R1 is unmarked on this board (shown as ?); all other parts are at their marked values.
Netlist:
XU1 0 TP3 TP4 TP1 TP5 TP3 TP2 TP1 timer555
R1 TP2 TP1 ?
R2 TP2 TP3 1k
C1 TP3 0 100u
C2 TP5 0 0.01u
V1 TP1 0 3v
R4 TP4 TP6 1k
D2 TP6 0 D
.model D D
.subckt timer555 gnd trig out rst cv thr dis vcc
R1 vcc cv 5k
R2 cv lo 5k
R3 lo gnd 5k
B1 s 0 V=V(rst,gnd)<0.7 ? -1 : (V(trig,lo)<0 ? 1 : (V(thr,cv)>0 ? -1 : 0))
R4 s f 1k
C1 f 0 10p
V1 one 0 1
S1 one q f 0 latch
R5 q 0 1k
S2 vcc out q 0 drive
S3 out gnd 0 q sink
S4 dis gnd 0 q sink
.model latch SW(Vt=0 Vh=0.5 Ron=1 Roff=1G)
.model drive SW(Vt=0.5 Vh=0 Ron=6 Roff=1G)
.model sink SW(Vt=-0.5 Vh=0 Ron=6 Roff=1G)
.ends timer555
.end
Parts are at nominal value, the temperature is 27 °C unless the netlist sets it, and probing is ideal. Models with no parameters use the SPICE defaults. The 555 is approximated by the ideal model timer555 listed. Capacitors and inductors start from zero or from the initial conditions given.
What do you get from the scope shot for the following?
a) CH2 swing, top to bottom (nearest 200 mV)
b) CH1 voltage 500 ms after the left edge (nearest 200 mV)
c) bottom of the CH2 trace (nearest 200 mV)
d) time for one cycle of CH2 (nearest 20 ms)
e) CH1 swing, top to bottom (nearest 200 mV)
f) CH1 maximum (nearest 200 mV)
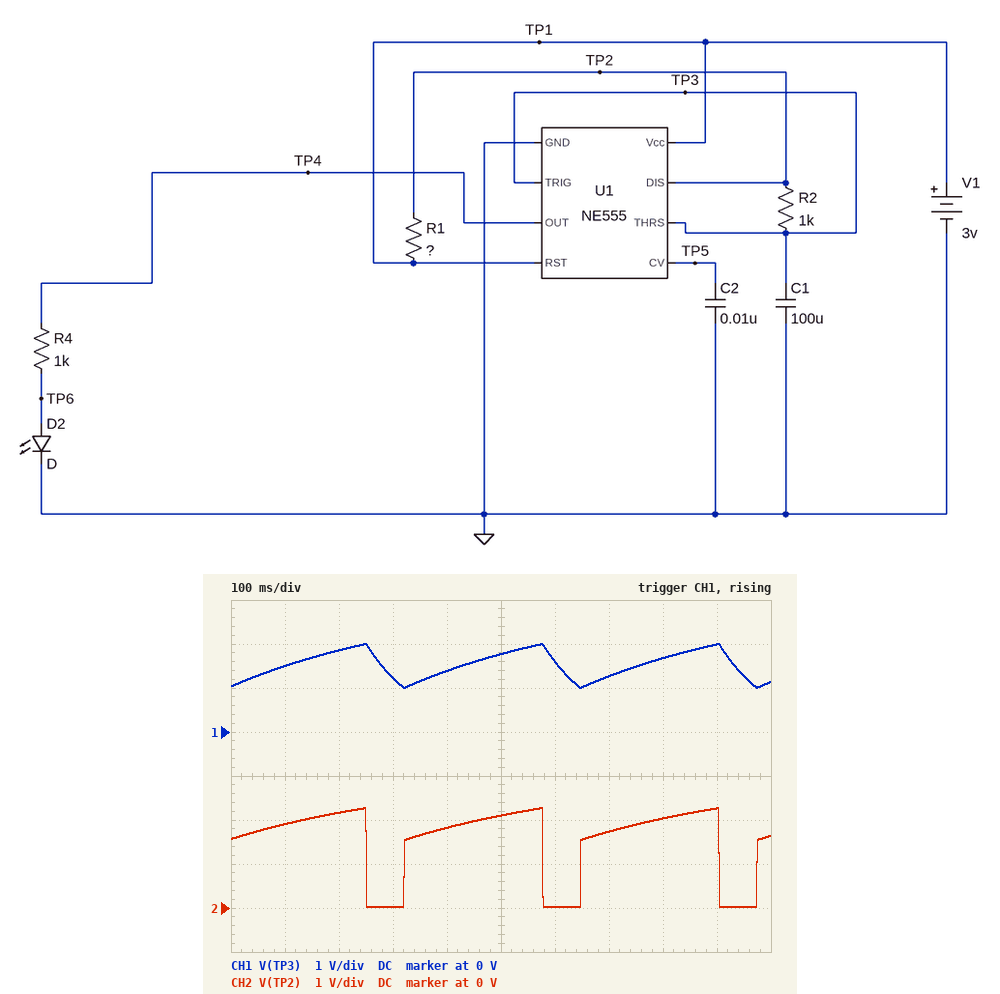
2.2 V
1.8 V
0 V
320 ms
1.0 V
2.0 V
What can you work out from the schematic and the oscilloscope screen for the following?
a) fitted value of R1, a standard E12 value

2.7 kΩ
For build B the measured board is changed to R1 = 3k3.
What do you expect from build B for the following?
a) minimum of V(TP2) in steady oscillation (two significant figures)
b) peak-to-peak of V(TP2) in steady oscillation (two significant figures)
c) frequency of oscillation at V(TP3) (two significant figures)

11 mV
2.2 V
2.7 Hz
